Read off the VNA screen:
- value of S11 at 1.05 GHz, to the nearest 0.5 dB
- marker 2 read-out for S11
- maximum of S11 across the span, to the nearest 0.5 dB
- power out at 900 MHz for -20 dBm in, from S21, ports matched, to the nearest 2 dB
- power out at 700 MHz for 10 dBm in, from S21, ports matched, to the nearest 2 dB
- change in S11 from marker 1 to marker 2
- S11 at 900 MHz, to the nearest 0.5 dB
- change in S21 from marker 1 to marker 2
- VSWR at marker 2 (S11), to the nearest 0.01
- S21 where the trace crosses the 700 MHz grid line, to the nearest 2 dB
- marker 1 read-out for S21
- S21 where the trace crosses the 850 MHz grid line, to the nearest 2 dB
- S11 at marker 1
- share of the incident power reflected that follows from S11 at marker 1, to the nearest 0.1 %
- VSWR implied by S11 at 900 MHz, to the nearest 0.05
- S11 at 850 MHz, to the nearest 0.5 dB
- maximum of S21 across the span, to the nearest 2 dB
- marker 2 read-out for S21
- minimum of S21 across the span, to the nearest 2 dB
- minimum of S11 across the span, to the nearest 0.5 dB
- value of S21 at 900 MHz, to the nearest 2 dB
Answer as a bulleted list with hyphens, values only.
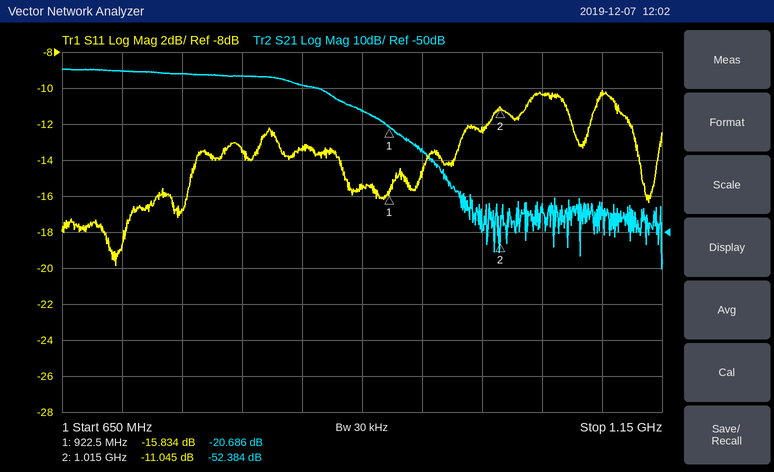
- -10.5 dB
- -11.045 dB
- -10.0 dB
- -36 dBm
- 4 dBm
- 4.789 dB
- -15.5 dB
- -31.698 dB
- 1.78
- -6 dB
- -20.686 dB
- -10 dB
- -15.834 dB
- 2.6 %
- 1.40
- -13.5 dB
- -4 dB
- -52.384 dB
- -60 dB
- -20.0 dB
- -16 dB
